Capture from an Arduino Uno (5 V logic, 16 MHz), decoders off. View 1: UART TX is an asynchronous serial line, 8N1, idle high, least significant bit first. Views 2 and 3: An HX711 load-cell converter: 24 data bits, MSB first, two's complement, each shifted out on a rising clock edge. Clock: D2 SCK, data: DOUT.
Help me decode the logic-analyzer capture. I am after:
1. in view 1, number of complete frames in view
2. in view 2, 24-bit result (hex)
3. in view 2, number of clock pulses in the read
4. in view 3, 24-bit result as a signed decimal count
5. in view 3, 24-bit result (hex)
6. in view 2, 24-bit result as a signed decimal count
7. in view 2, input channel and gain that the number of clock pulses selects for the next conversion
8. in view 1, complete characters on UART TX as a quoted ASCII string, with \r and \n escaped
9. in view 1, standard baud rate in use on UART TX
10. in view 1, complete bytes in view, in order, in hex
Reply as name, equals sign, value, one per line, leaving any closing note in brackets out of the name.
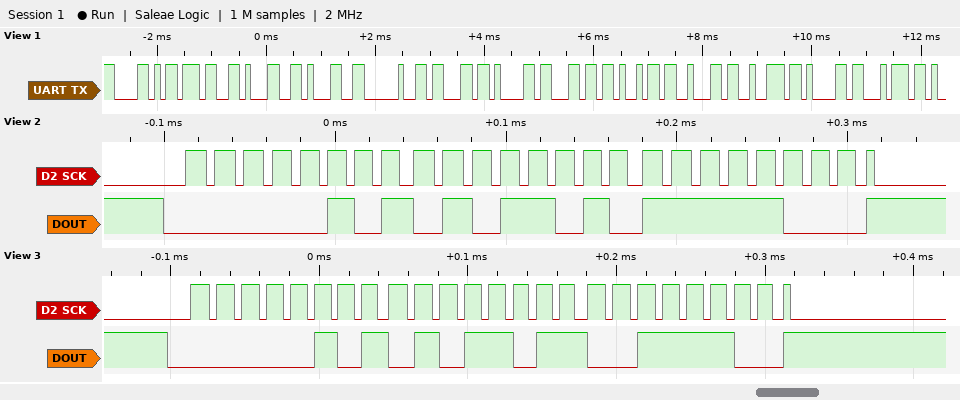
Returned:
in view 1, number of complete frames in view = 13
in view 2, 24-bit result = 0x055AF8
in view 2, number of clock pulses in the read = 25
in view 3, 24-bit result as a signed decimal count = 351036
in view 3, 24-bit result = 0x055B3C
in view 2, 24-bit result as a signed decimal count = 350968
in view 2, input channel and gain that the number of clock pulses selects for the next conversion = channel A, gain 128
in view 1, complete characters on UART TX as a quoted ASCII string, with \r and \n escaped = "X711 calibrat"
in view 1, standard baud rate in use on UART TX = 9600 baud
in view 1, complete bytes in view, in order, in hex = 58 37 31 31 20 63 61 6C 69 62 72 61 74
